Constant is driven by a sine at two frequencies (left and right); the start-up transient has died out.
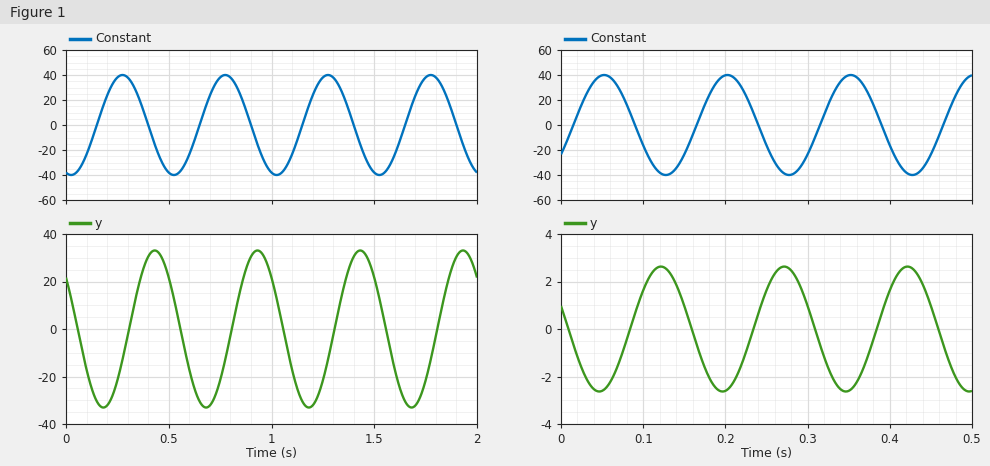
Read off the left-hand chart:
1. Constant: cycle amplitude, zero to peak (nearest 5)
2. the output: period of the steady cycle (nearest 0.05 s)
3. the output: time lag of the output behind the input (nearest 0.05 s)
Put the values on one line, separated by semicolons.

40; 0.50 s; 0.15 s
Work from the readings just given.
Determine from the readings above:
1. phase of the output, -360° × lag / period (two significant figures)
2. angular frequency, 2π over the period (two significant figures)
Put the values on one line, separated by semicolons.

-110°; 13 rad/s
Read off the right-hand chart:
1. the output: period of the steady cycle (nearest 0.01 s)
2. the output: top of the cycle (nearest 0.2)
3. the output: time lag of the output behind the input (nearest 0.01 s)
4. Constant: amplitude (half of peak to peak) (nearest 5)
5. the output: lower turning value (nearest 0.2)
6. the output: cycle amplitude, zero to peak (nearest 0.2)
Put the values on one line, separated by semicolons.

0.15 s; 2.6; 0.07 s; 40; -2.6; 2.6
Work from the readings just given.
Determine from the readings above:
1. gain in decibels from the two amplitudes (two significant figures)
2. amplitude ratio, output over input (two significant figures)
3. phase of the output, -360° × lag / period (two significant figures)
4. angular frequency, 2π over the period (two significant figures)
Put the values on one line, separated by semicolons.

-24 dB; 0.065; -170°; 42 rad/s
